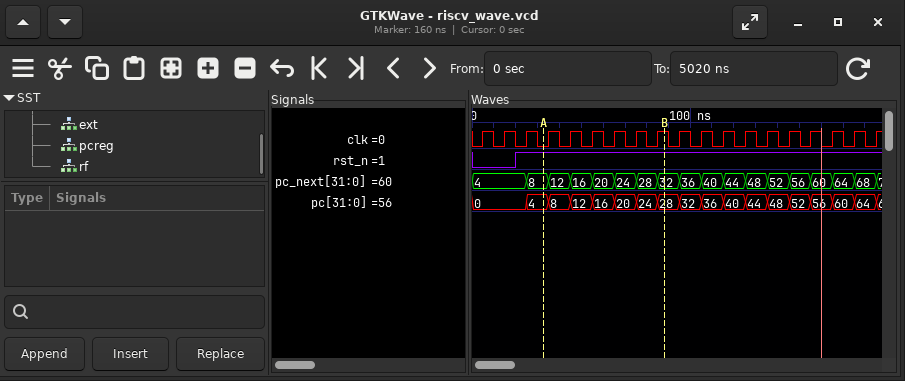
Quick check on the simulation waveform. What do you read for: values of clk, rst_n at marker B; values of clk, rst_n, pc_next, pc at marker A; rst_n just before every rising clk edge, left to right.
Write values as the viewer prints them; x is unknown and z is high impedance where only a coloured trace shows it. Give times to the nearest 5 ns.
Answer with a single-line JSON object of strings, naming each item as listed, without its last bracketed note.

{"values of clk, rst_n at marker B": "clk=1, rst_n=1", "values of clk, rst_n, pc_next, pc at marker A": "clk=0, rst_n=1, pc_next=8, pc=4", "rst_n just before every rising clk edge, left to right": "0 0 1 1 1 1 1 1 1 1 1 1 1 1 1 1 1 1 1"}
